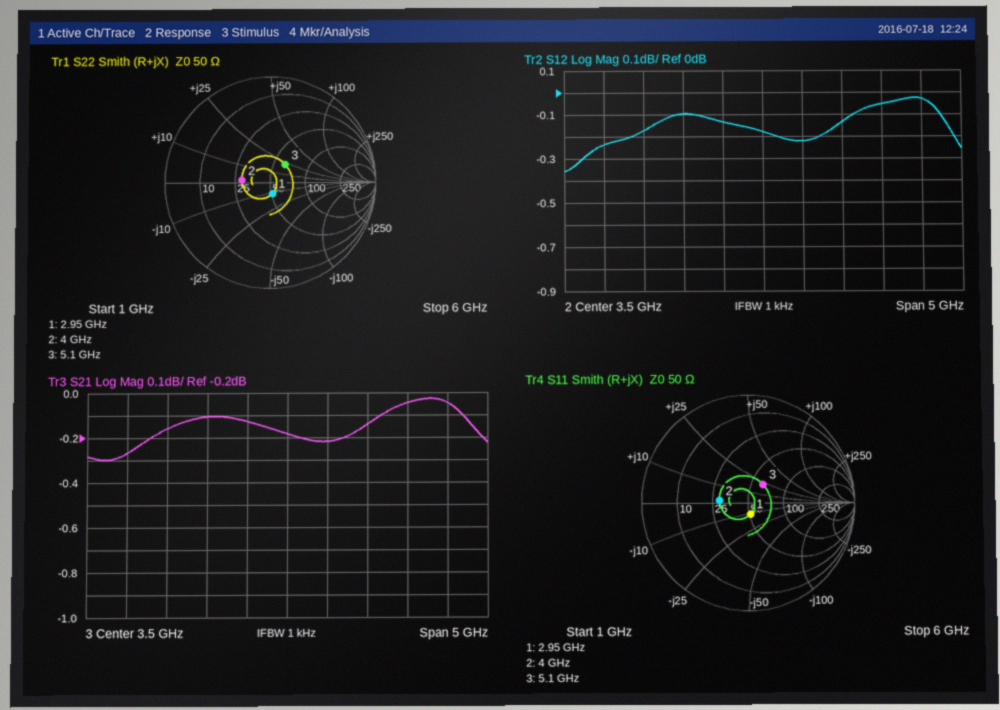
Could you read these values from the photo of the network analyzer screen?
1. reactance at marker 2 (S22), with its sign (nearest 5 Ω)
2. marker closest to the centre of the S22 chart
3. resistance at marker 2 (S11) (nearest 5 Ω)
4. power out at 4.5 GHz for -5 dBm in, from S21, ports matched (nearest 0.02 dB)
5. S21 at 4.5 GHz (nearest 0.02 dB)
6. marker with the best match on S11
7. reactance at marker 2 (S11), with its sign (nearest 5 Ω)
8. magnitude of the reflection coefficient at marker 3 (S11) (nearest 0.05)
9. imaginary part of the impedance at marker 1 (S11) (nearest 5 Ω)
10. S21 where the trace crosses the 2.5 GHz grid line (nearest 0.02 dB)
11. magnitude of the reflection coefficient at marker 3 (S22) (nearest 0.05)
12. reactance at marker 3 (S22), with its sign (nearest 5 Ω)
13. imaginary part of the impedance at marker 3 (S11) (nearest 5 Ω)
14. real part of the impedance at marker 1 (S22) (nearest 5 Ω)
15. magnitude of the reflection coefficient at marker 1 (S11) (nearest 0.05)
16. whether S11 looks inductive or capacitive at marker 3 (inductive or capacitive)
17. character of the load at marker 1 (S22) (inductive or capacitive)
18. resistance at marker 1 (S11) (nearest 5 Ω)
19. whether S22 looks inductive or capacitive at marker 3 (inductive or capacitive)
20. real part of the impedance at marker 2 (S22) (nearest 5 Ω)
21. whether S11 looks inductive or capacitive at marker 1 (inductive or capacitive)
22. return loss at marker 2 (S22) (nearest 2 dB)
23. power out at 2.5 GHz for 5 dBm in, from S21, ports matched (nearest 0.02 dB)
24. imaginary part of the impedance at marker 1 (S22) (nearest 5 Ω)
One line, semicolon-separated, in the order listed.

0 Ω; marker 1; 30 Ω; -5.14 dBm; -0.14 dB; marker 1; 0 Ω; 0.20; -10 Ω; -0.10 dB; 0.20; +20 Ω; +20 Ω; 50 Ω; 0.10; inductive; capacitive; 50 Ω; inductive; 30 Ω; capacitive; 12 dB; 4.90 dBm; -10 Ω
